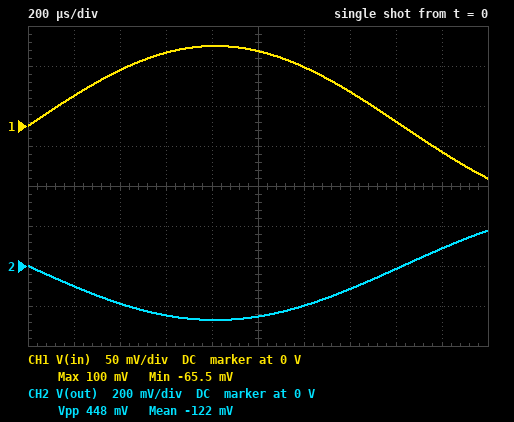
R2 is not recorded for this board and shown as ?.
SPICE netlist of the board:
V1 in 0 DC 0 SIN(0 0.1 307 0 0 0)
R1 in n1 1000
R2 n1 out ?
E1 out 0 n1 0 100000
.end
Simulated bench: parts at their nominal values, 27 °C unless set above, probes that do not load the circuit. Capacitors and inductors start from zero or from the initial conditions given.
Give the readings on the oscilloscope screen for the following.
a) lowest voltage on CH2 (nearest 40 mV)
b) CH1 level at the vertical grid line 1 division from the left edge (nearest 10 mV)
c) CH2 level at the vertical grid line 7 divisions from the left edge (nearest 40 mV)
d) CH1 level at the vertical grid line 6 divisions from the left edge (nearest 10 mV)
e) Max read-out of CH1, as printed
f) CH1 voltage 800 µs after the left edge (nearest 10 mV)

-280 mV
40 mV
-120 mV
70 mV
100 mV
100 mV
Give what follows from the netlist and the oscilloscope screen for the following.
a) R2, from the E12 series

2.7 kΩ
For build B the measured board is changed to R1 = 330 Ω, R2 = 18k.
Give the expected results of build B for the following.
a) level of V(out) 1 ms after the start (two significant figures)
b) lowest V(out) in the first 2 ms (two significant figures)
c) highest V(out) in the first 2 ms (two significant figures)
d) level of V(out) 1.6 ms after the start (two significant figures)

-5.1 V
-5.5 V
3.6 V
-300 mV
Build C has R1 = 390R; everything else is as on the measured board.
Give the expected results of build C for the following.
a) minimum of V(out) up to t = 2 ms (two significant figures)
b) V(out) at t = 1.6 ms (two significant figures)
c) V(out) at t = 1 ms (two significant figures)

-690 mV
-38 mV
-650 mV
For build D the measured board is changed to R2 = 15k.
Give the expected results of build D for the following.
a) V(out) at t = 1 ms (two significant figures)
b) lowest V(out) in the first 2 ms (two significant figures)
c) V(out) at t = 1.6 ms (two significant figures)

-1.4 V
-1.5 V
-83 mV
